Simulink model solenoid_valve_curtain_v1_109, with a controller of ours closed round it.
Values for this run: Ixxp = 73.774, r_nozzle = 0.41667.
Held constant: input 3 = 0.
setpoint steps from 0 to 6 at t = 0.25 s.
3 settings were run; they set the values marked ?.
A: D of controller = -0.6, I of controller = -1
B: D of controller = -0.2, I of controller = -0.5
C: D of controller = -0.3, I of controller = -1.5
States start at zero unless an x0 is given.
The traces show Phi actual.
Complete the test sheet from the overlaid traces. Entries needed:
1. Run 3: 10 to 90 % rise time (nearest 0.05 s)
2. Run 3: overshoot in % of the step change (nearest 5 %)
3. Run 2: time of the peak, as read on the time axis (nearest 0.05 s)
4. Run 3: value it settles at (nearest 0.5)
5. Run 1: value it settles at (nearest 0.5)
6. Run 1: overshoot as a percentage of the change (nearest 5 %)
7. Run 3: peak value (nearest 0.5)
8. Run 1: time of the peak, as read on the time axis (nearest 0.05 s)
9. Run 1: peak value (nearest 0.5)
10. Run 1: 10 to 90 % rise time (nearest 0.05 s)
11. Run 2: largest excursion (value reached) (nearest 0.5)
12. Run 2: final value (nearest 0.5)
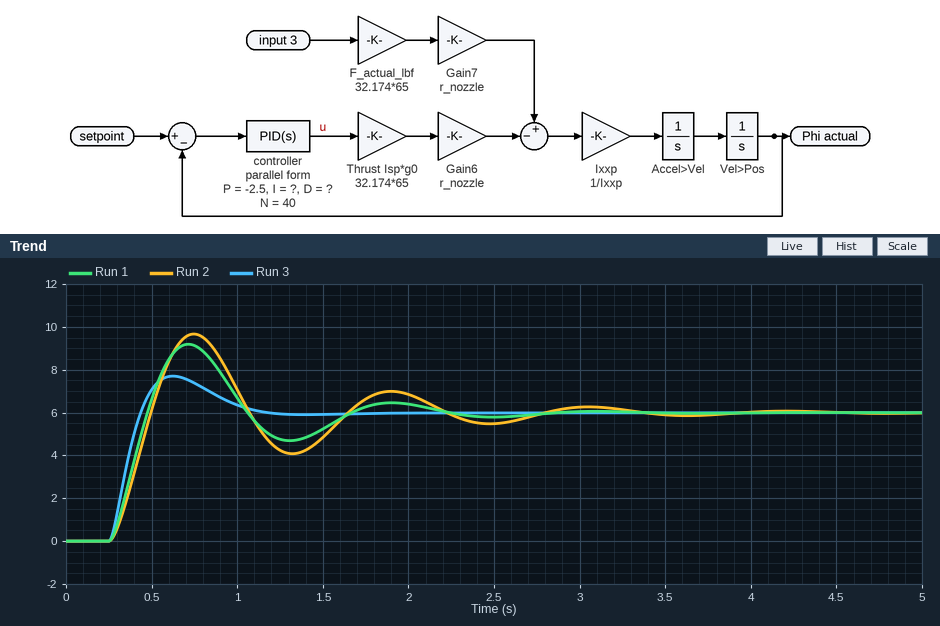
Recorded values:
0.15 s
30 %
0.75 s
6.0
6.0
55 %
7.5
0.70 s
9.0
0.15 s
9.5
6.0
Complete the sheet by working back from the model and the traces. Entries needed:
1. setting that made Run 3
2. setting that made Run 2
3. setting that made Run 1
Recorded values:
A
B
C
